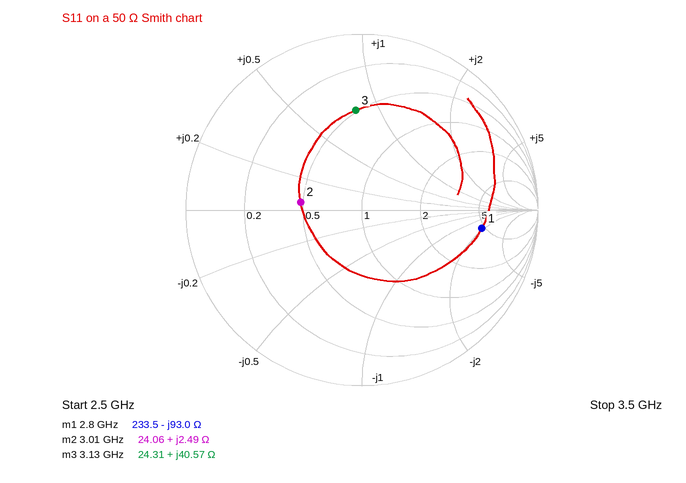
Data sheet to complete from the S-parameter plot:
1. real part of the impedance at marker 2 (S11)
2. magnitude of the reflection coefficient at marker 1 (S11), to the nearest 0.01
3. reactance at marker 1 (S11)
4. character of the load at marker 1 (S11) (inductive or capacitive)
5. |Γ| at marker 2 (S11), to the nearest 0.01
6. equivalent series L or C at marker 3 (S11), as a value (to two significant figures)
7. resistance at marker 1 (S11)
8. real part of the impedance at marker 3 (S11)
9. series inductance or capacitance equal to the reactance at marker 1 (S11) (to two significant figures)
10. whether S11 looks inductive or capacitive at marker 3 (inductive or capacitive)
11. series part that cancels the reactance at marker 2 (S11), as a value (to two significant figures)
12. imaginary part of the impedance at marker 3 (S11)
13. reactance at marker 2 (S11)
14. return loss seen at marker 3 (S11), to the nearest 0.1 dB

24.06 Ω
0.69
-93.0 Ω
capacitive
0.35
2.1 nH
233.5 Ω
24.31 Ω
610 fF
inductive
21 pF
+40.57 Ω
+2.49 Ω
4.9 dB
